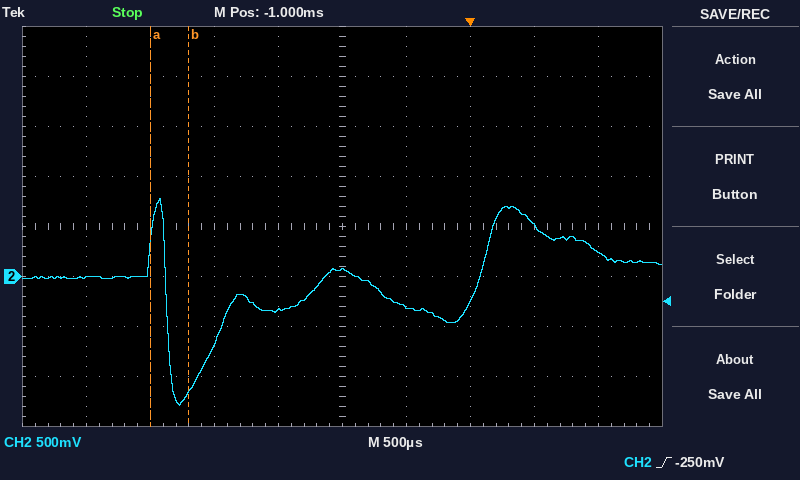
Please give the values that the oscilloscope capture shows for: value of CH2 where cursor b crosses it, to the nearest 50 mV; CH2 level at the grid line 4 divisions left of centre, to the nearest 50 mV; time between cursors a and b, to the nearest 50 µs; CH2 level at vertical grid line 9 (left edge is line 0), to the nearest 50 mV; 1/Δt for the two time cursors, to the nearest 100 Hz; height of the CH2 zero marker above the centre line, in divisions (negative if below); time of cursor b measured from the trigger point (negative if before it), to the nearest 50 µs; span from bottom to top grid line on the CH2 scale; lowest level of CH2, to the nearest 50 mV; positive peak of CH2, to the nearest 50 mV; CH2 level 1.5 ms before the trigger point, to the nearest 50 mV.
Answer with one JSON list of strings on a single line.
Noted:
["-1.15 V", "0 mV", "300 µs", "250 mV", "3.3 kHz", "-1.0 div", "-2.20 ms", "4 V", "-1.30 V", "800 mV", "-350 mV"]
